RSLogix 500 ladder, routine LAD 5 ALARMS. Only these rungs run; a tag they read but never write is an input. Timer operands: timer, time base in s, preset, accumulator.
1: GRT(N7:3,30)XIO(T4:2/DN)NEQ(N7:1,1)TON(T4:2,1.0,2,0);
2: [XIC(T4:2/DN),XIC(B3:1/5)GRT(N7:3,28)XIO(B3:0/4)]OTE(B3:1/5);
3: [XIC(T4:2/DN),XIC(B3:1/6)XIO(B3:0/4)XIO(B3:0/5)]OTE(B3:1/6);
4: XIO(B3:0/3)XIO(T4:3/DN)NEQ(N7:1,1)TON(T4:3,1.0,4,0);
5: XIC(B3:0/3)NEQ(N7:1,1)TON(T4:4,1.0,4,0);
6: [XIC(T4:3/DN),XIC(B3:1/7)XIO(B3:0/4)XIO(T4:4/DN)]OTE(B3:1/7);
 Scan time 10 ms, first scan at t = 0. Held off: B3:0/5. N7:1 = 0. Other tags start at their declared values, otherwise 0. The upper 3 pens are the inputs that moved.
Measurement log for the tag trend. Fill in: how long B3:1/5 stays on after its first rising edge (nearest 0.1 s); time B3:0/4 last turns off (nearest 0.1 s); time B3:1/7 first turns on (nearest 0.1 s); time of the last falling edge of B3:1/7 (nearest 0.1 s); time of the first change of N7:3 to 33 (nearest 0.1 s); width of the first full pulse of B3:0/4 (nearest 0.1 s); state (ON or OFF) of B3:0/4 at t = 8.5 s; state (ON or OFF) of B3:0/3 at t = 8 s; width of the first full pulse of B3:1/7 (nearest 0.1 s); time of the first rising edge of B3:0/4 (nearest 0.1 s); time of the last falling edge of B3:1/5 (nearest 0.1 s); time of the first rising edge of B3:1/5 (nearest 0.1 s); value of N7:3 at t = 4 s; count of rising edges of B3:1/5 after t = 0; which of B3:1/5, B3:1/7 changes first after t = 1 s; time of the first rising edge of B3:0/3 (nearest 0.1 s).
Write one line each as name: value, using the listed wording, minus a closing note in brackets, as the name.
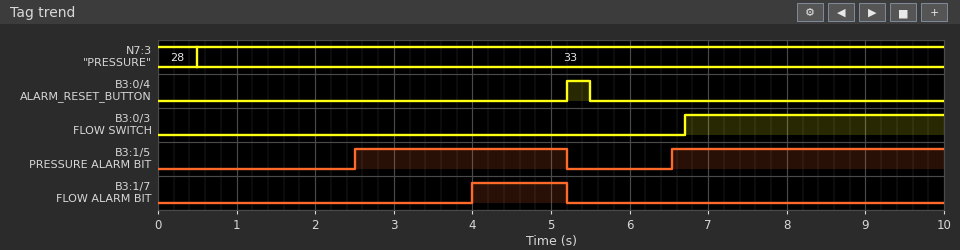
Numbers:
how long B3:1/5 stays on after its first rising edge: 2.7 s
time B3:0/4 last turns off: 5.5 s
time B3:1/7 first turns on: 4.0 s
time of the last falling edge of B3:1/7: 5.2 s
time of the first change of N7:3 to 33: 0.5 s
width of the first full pulse of B3:0/4: 0.3 s
state (ON or OFF) of B3:0/4 at t = 8.5 s: OFF
state (ON or OFF) of B3:0/3 at t = 8 s: ON
width of the first full pulse of B3:1/7: 1.2 s
time of the first rising edge of B3:0/4: 5.2 s
time of the last falling edge of B3:1/5: 5.2 s
time of the first rising edge of B3:1/5: 2.5 s
value of N7:3 at t = 4 s: 33
count of rising edges of B3:1/5 after t = 0: 2
which of B3:1/5, B3:1/7 changes first after t = 1 s: B3:1/5
time of the first rising edge of B3:0/3: 6.7 s
